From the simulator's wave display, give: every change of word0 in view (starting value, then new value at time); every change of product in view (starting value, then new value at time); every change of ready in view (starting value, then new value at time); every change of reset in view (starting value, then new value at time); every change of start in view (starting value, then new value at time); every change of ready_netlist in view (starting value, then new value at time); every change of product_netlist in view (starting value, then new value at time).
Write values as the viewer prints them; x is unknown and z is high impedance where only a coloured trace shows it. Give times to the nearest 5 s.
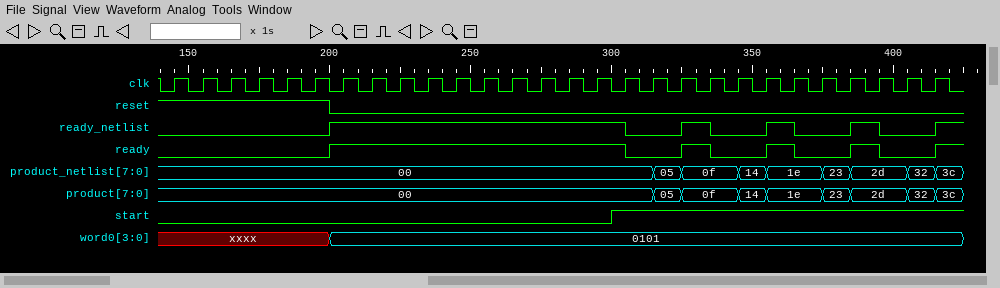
xxxx, 0101 at 200 s
00, 05 at 315 s, 0f at 325 s, 14 at 345 s, 1e at 355 s, 23 at 375 s, 2d at 385 s, 32 at 405 s, 3c at 415 s
0, 1 at 200 s, 0 at 305 s, 1 at 325 s, 0 at 335 s, 1 at 355 s, 0 at 365 s, 1 at 385 s, 0 at 395 s, 1 at 415 s
1, 0 at 200 s
0, 1 at 300 s
0, 1 at 200 s, 0 at 305 s, 1 at 325 s, 0 at 335 s, 1 at 355 s, 0 at 365 s, 1 at 385 s, 0 at 395 s, 1 at 415 s
00, 05 at 315 s, 0f at 325 s, 14 at 345 s, 1e at 355 s, 23 at 375 s, 2d at 385 s, 32 at 405 s, 3c at 415 s
